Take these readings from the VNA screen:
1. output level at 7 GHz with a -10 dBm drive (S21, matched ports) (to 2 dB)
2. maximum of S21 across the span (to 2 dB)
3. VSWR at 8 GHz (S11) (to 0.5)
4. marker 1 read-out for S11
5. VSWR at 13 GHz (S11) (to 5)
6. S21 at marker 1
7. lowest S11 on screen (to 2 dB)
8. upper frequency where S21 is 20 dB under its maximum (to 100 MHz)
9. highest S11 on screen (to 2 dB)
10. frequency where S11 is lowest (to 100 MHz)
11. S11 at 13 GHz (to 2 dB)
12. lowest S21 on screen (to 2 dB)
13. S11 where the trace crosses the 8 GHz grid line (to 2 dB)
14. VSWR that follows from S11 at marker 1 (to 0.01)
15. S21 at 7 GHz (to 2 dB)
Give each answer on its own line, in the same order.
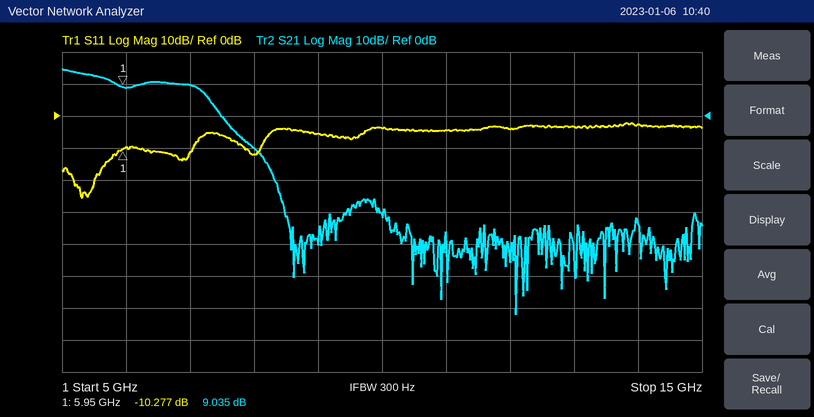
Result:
0 dBm
14 dB
1.5
-10.277 dB
5
9.035 dB
-26 dB
7.7 GHz
-2 dB
5.3 GHz
-4 dB
-62 dB
-12 dB
1.88
10 dB
